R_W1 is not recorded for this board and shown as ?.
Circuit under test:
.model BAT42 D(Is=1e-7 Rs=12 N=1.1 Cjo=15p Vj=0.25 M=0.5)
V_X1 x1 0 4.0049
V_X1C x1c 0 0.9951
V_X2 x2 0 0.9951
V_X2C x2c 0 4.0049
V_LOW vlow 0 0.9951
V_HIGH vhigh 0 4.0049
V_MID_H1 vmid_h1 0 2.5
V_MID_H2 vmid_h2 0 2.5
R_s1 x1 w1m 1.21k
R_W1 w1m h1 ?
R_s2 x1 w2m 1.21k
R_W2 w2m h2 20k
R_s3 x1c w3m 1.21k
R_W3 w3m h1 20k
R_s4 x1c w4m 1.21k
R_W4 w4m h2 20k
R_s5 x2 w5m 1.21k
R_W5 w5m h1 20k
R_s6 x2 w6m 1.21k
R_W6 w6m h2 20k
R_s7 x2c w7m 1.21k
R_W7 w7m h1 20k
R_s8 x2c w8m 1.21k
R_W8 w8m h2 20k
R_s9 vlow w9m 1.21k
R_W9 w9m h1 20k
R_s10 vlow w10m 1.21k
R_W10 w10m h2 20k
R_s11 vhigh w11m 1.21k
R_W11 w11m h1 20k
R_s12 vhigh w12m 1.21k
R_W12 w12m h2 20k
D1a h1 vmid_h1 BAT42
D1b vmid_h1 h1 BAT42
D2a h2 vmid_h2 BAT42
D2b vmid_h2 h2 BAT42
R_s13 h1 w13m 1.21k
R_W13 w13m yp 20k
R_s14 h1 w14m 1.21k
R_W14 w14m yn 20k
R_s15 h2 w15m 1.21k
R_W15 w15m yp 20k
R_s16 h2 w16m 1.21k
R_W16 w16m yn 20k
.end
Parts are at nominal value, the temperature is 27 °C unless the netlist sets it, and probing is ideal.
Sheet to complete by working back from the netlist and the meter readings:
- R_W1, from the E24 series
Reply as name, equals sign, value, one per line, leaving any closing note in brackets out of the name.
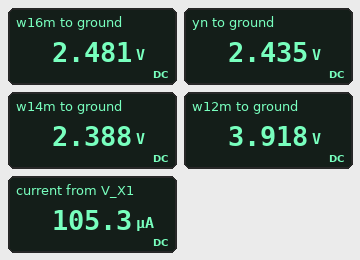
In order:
R_W1, from the E24 series = 47 kΩ
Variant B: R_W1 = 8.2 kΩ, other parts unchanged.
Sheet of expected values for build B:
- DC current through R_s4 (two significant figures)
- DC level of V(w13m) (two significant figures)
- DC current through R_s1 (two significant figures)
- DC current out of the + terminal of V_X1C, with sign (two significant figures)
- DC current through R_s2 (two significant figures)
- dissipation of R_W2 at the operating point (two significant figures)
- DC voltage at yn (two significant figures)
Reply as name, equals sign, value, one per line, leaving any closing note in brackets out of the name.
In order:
DC current through R_s4 = 72 µA
DC level of V(w13m) = 2.7 V
DC current through R_s1 = 140 µA
DC current out of the + terminal of V_X1C, with sign = -150 µA
DC current through R_s2 = 70 µA
dissipation of R_W2 at the operating point = 98 µW
DC voltage at yn = 2.6 V
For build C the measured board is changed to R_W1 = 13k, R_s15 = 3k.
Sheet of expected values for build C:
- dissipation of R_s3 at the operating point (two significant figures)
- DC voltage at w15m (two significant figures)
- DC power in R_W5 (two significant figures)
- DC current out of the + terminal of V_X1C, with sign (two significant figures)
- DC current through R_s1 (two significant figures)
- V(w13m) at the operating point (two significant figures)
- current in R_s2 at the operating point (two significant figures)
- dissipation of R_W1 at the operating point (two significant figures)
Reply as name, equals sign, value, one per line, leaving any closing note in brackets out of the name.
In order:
dissipation of R_s3 at the operating point = 6.9 µW
DC voltage at w15m = 2.5 V
DC power in R_W5 = 110 µW
DC current out of the + terminal of V_X1C, with sign = -150 µA
DC current through R_s1 = 99 µA
V(w13m) at the operating point = 2.6 V
current in R_s2 at the operating point = 70 µA
dissipation of R_W1 at the operating point = 130 µW
